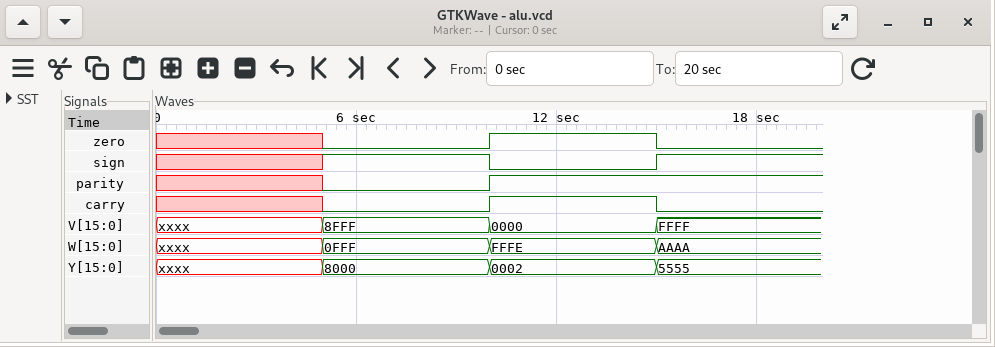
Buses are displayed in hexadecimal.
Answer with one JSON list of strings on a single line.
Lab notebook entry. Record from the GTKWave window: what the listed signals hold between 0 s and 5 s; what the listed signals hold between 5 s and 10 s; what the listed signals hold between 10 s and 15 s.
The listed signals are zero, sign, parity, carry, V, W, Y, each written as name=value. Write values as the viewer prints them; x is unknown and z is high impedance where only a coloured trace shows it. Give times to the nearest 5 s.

["zero=x, sign=x, parity=x, carry=x, V=xxxx, W=xxxx, Y=xxxx", "zero=0, sign=1, parity=0, carry=0, V=8FFF, W=0FFF, Y=8000", "zero=1, sign=0, parity=1, carry=1, V=0000, W=FFFE, Y=0002"]
